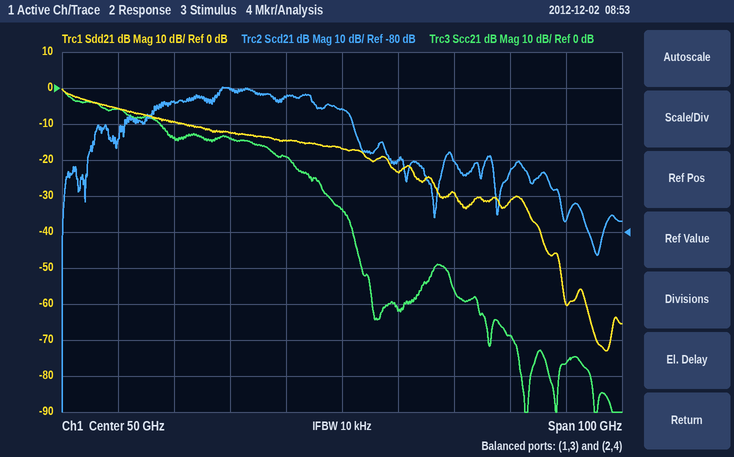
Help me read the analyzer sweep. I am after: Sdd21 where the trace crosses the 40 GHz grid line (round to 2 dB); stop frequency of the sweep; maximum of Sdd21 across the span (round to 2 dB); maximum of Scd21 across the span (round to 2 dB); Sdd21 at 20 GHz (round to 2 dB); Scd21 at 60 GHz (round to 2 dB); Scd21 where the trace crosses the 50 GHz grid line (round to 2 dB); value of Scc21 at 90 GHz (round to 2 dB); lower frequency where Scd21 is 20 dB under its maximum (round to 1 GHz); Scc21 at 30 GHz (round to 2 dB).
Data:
-14 dB
100 GHz
0 dB
-40 dB
-10 dB
-60 dB
-46 dB
-76 dB
5 GHz
-14 dB
